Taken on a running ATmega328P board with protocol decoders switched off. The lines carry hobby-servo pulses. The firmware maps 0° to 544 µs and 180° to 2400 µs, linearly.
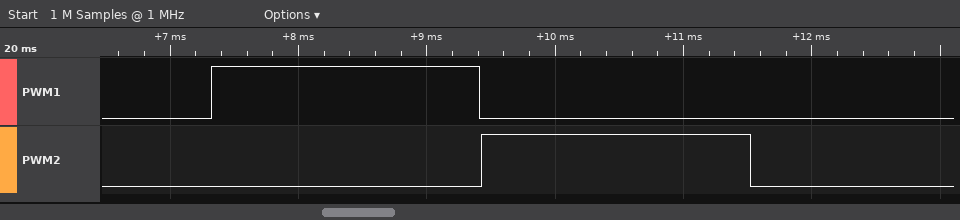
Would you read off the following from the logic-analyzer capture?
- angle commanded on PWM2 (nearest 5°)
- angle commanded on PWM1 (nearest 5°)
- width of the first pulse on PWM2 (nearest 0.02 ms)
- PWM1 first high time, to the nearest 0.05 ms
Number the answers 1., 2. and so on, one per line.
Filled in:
1. 150°
2. 150°
3. 2.10 ms
4. 2.10 ms
